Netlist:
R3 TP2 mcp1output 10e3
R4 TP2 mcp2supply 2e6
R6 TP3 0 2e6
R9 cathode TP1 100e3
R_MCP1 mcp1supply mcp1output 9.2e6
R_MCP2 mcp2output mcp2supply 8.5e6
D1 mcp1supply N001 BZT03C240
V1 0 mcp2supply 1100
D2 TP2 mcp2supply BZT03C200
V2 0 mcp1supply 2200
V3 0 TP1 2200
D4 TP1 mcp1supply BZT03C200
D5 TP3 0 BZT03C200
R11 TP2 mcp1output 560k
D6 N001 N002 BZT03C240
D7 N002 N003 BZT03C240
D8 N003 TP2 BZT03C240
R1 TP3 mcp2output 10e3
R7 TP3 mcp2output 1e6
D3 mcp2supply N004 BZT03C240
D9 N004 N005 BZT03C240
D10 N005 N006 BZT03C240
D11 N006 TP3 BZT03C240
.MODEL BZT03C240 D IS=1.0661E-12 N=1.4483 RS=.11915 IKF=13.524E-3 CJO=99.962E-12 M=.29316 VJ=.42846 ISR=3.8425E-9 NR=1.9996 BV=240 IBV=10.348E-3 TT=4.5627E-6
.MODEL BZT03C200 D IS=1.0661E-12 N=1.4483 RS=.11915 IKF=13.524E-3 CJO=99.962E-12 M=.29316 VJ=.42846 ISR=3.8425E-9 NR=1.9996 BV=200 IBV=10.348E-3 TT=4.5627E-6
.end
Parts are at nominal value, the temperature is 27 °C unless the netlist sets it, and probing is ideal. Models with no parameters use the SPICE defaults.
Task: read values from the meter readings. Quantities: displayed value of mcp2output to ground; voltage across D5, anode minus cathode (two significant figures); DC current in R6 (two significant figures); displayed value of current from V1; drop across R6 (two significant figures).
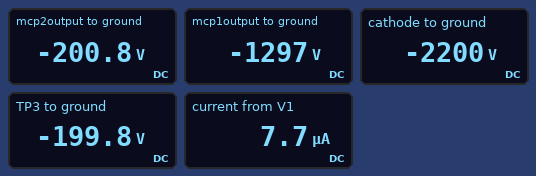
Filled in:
-200.8 V
-200 V
100 µA
7.7 µA
200 V
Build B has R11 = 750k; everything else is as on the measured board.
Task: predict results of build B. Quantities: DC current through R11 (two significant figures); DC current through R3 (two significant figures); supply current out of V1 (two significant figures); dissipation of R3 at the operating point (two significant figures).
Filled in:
1.3 µA
97 µA
7.7 µA
94 µW
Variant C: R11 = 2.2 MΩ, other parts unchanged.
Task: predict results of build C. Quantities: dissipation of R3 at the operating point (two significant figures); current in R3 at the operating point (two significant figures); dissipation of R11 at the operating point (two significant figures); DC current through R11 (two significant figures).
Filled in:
95 µW
98 µA
430 nW
440 nA
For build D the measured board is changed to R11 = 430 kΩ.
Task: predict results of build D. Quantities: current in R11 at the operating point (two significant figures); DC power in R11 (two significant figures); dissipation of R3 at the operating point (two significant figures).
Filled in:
2.2 µA
2.1 µW
92 µW
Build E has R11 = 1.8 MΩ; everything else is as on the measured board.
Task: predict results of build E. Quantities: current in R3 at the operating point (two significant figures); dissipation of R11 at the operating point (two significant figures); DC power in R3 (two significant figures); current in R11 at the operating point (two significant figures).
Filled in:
98 µA
530 nW
95 µW
540 nA
